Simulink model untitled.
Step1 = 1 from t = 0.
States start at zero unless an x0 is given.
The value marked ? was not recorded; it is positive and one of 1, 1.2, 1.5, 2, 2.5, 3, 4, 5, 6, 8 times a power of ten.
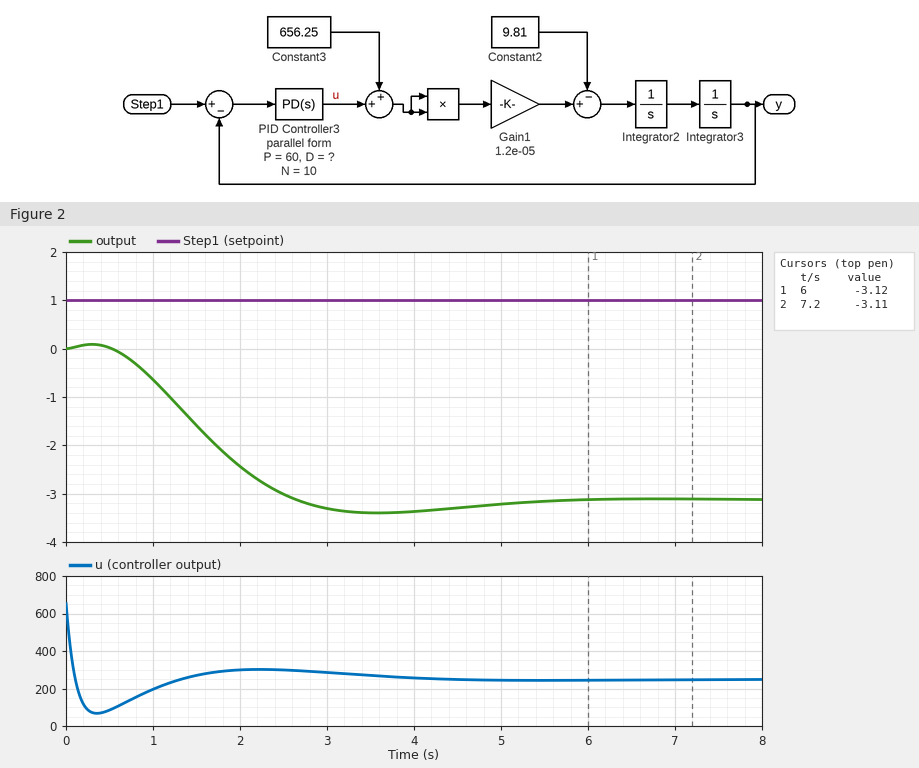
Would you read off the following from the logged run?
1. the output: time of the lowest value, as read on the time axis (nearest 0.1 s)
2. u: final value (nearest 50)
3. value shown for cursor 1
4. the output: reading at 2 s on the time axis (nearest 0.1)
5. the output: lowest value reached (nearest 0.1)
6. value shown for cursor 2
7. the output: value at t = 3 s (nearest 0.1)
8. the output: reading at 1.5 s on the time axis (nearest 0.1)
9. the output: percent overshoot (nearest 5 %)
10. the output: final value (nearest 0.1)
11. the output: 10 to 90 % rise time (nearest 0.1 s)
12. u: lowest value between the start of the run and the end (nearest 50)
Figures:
3.6 s
250
-3.12
-2.4
-3.4
-3.11
-3.3
-1.6
10 %
-3.1
1.5 s
50
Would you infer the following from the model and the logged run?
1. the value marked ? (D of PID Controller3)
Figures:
60
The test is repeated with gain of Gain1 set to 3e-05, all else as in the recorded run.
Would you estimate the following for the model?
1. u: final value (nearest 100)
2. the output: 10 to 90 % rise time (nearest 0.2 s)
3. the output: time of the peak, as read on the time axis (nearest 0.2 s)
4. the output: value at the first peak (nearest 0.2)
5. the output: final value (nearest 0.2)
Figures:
-100
0.8 s
1.8 s
2.6
2.4
